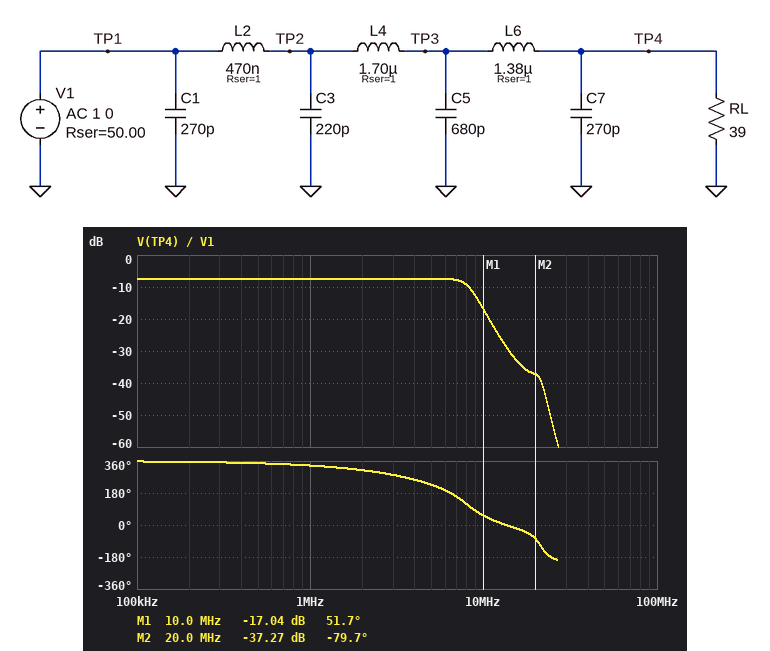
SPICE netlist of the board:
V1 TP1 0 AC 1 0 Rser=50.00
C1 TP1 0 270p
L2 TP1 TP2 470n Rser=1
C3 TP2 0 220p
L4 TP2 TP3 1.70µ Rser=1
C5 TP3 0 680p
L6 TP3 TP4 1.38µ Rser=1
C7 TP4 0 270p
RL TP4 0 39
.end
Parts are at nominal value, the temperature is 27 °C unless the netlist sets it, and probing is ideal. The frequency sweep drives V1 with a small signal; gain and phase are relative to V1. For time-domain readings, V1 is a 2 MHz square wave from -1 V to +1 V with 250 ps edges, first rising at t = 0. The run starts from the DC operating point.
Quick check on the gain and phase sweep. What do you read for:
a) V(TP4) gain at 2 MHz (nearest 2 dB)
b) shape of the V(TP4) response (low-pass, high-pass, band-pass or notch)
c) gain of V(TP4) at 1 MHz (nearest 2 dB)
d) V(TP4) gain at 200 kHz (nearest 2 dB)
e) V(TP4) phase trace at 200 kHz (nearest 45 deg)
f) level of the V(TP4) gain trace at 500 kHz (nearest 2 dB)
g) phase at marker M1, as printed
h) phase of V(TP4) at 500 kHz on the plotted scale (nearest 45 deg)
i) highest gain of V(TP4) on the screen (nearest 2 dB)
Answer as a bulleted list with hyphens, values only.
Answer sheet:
- -8 dB
- low-pass
- -8 dB
- -8 dB
- 360 deg
- -8 dB
- 51.7 deg
- 360 deg
- -8 dB
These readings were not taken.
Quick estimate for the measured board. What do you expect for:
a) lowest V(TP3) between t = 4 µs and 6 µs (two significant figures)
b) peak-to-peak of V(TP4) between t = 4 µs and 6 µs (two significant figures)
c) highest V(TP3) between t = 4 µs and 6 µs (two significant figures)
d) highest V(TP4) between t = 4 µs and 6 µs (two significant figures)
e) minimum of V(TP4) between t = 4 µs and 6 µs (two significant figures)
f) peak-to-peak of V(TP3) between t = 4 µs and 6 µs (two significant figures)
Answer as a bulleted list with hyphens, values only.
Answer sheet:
- -660 mV
- 1.1 V
- 660 mV
- 530 mV
- -530 mV
- 1.3 V
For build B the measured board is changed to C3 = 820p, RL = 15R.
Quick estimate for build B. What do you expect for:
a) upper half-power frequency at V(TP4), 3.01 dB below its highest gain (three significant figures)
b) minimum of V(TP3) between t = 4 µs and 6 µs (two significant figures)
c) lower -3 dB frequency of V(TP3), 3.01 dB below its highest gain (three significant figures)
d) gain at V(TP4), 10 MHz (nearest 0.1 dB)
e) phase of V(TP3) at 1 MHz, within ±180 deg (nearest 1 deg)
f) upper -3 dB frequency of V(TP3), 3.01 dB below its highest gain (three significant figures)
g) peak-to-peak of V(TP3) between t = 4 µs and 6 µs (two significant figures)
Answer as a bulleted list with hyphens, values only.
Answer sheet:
- 7.99 MHz
- -700 mV
- 6.46 MHz
- -28.0 dB
- 0 deg
- 8.10 MHz
- 1.4 V
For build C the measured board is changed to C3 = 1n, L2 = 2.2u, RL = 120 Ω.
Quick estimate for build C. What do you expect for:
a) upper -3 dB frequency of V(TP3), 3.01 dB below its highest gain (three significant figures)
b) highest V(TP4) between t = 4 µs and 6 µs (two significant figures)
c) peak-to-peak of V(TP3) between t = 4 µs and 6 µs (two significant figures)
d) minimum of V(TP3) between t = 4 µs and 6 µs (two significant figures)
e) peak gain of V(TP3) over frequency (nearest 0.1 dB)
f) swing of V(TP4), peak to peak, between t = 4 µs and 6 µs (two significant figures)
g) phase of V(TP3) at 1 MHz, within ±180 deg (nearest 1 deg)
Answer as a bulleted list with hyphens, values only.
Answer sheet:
- 5.63 MHz
- 890 mV
- 1.5 V
- -740 mV
- -3.1 dB
- 1.8 V
- -36 deg
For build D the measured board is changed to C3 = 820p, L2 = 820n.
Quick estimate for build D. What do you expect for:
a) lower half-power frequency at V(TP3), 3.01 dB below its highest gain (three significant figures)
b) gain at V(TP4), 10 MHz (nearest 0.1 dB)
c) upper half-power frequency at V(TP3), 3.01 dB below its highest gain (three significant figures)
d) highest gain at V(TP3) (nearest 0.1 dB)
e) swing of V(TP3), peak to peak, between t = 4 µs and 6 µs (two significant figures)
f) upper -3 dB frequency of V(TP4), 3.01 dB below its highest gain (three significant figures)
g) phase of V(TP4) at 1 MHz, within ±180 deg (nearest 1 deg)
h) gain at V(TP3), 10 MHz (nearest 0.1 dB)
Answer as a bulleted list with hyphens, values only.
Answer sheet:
- 2.79 MHz
- -18.2 dB
- 8.94 MHz
- -3.6 dB
- 1.3 V
- 8.41 MHz
- -32 deg
- -11.0 dB
